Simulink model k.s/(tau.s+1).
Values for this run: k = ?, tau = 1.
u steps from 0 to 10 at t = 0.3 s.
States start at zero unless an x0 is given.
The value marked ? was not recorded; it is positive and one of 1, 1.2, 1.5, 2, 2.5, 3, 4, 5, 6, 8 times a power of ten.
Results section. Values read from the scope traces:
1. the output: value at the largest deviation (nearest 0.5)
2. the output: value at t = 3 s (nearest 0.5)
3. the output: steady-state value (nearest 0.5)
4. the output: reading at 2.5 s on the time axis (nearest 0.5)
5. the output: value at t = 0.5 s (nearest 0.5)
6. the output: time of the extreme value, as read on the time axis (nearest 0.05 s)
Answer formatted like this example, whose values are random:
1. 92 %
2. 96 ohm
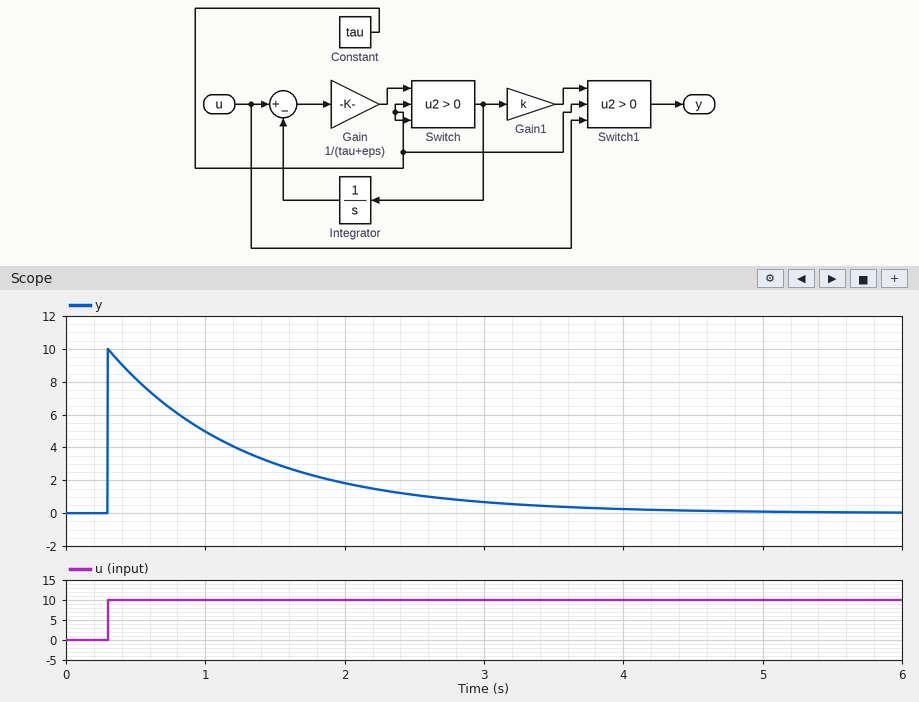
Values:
1. 10.0
2. 0.5
3. 0.0
4. 1.0
5. 8.0
6. 0.30 s
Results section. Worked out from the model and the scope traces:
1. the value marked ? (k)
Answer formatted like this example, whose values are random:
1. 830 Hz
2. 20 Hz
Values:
1. 1
